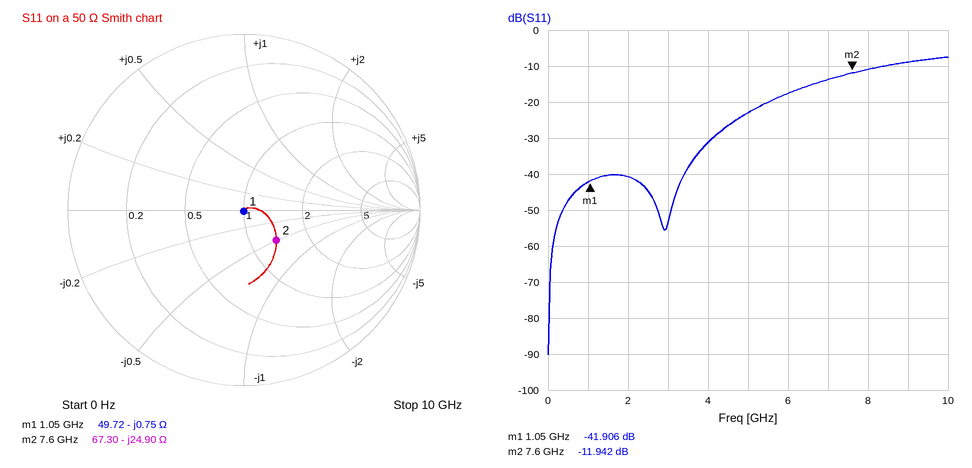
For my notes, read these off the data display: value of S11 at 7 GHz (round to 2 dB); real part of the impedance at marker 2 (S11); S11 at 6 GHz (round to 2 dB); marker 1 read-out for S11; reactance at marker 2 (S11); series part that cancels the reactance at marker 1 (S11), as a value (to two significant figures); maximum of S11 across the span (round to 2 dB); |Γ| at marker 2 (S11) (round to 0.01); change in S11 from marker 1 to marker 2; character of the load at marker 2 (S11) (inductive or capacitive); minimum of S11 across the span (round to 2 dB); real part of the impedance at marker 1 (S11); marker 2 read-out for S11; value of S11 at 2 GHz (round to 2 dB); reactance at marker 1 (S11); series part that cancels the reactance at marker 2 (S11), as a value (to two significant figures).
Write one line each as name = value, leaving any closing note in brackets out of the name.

value of S11 at 7 GHz = -14 dB
real part of the impedance at marker 2 = 67.30 Ω
S11 at 6 GHz = -18 dB
marker 1 read-out for S11 = -41.906 dB
reactance at marker 2 = -24.90 Ω
series part that cancels the reactance at marker 1 (S11), as a value = 110 pH
maximum of S11 across the span = -8 dB
|Γ| at marker 2 (S11) = 0.25
change in S11 from marker 1 to marker 2 = 29.964 dB
character of the load at marker 2 (S11) = capacitive
minimum of S11 across the span = -90 dB
real part of the impedance at marker 1 = 49.72 Ω
marker 2 read-out for S11 = -11.942 dB
value of S11 at 2 GHz = -40 dB
reactance at marker 1 = -0.75 Ω
series part that cancels the reactance at marker 2 (S11), as a value = 520 pH
